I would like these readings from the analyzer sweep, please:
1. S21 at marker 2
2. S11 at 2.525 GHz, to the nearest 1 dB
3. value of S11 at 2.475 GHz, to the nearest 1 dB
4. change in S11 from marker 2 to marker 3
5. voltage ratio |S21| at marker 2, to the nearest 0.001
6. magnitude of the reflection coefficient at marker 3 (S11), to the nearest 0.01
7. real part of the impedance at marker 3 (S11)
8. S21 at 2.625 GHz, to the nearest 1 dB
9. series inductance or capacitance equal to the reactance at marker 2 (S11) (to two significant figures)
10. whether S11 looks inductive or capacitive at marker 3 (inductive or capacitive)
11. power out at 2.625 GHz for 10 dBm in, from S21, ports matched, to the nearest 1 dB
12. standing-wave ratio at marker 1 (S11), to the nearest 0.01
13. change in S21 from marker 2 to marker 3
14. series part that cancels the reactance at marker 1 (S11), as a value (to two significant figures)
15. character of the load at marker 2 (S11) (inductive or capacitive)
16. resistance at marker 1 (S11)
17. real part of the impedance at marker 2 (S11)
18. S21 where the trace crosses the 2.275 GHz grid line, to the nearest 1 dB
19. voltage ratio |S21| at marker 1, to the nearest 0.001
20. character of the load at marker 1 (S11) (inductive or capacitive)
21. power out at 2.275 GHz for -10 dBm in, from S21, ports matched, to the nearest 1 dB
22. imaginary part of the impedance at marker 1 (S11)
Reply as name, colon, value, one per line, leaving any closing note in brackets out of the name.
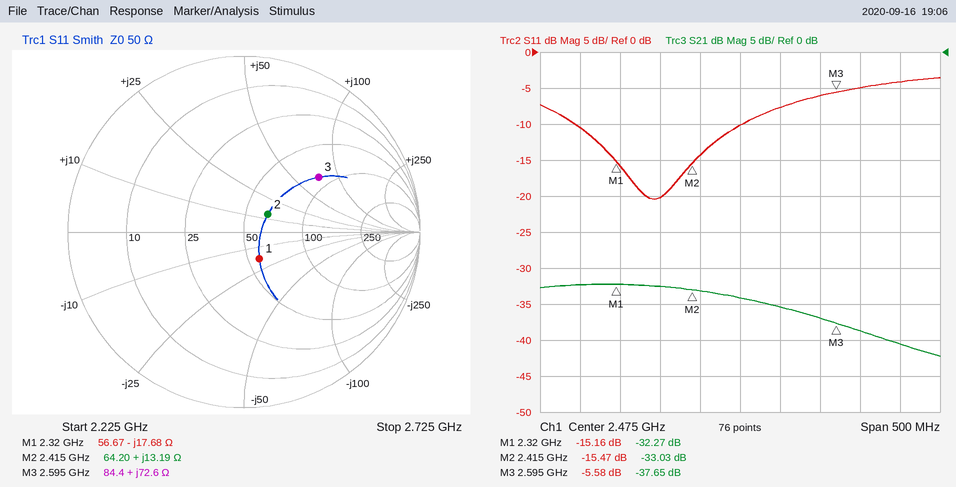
S21 at marker 2: -33.03 dB
S11 at 2.525 GHz, to the nearest 1 dB: -8 dB
value of S11 at 2.475 GHz, to the nearest 1 dB: -10 dB
change in S11 from marker 2 to marker 3: 9.89 dB
voltage ratio |S21| at marker 2, to the nearest 0.001: 0.022
magnitude of the reflection coefficient at marker 3 (S11), to the nearest 0.01: 0.53
real part of the impedance at marker 3: 84.4 Ω
S21 at 2.625 GHz, to the nearest 1 dB: -39 dB
series inductance or capacitance equal to the reactance at marker 2 (S11): 870 pH
whether S11 looks inductive or capacitive at marker 3: inductive
power out at 2.625 GHz for 10 dBm in, from S21, ports matched, to the nearest 1 dB: -29 dBm
standing-wave ratio at marker 1 (S11), to the nearest 0.01: 1.42
change in S21 from marker 2 to marker 3: -4.62 dB
series part that cancels the reactance at marker 1 (S11), as a value: 1.2 nH
character of the load at marker 2 (S11): inductive
resistance at marker 1: 56.67 Ω
real part of the impedance at marker 2: 64.20 Ω
S21 where the trace crosses the 2.275 GHz grid line, to the nearest 1 dB: -32 dB
voltage ratio |S21| at marker 1, to the nearest 0.001: 0.024
character of the load at marker 1 (S11): capacitive
power out at 2.275 GHz for -10 dBm in, from S21, ports matched, to the nearest 1 dB: -42 dBm
imaginary part of the impedance at marker 1: -17.68 Ω
